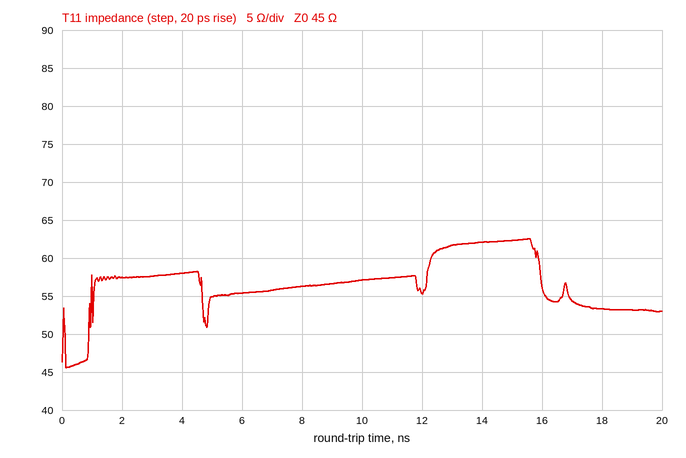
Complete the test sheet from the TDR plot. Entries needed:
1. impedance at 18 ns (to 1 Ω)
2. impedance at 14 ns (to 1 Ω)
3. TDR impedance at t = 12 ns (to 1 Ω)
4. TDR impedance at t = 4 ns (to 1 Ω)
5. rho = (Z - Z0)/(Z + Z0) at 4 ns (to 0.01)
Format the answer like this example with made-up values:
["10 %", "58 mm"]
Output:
["53 Ω", "62 Ω", "55 Ω", "58 Ω", "+0.13"]
